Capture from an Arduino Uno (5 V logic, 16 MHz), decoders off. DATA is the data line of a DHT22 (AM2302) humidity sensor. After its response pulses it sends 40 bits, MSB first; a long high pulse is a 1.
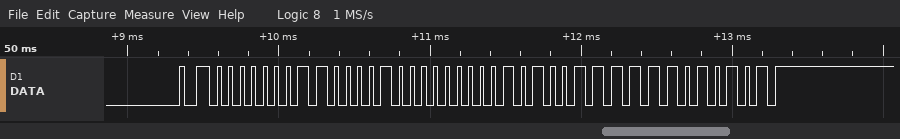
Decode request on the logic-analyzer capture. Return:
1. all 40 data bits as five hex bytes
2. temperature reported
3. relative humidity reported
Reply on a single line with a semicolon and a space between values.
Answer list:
01 84 01 4F D5; 33.5 °C; 38.8 %
